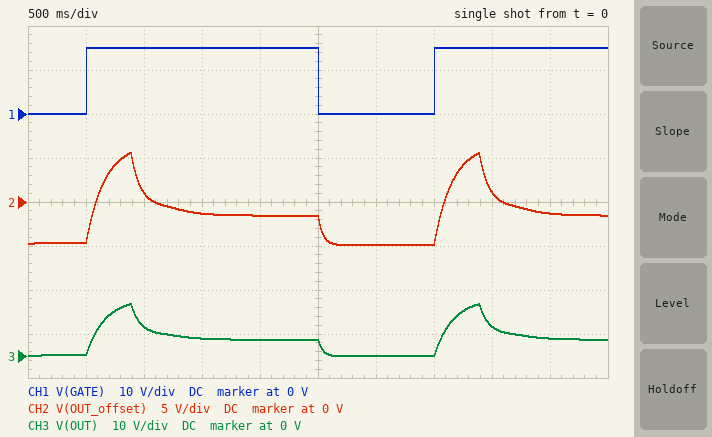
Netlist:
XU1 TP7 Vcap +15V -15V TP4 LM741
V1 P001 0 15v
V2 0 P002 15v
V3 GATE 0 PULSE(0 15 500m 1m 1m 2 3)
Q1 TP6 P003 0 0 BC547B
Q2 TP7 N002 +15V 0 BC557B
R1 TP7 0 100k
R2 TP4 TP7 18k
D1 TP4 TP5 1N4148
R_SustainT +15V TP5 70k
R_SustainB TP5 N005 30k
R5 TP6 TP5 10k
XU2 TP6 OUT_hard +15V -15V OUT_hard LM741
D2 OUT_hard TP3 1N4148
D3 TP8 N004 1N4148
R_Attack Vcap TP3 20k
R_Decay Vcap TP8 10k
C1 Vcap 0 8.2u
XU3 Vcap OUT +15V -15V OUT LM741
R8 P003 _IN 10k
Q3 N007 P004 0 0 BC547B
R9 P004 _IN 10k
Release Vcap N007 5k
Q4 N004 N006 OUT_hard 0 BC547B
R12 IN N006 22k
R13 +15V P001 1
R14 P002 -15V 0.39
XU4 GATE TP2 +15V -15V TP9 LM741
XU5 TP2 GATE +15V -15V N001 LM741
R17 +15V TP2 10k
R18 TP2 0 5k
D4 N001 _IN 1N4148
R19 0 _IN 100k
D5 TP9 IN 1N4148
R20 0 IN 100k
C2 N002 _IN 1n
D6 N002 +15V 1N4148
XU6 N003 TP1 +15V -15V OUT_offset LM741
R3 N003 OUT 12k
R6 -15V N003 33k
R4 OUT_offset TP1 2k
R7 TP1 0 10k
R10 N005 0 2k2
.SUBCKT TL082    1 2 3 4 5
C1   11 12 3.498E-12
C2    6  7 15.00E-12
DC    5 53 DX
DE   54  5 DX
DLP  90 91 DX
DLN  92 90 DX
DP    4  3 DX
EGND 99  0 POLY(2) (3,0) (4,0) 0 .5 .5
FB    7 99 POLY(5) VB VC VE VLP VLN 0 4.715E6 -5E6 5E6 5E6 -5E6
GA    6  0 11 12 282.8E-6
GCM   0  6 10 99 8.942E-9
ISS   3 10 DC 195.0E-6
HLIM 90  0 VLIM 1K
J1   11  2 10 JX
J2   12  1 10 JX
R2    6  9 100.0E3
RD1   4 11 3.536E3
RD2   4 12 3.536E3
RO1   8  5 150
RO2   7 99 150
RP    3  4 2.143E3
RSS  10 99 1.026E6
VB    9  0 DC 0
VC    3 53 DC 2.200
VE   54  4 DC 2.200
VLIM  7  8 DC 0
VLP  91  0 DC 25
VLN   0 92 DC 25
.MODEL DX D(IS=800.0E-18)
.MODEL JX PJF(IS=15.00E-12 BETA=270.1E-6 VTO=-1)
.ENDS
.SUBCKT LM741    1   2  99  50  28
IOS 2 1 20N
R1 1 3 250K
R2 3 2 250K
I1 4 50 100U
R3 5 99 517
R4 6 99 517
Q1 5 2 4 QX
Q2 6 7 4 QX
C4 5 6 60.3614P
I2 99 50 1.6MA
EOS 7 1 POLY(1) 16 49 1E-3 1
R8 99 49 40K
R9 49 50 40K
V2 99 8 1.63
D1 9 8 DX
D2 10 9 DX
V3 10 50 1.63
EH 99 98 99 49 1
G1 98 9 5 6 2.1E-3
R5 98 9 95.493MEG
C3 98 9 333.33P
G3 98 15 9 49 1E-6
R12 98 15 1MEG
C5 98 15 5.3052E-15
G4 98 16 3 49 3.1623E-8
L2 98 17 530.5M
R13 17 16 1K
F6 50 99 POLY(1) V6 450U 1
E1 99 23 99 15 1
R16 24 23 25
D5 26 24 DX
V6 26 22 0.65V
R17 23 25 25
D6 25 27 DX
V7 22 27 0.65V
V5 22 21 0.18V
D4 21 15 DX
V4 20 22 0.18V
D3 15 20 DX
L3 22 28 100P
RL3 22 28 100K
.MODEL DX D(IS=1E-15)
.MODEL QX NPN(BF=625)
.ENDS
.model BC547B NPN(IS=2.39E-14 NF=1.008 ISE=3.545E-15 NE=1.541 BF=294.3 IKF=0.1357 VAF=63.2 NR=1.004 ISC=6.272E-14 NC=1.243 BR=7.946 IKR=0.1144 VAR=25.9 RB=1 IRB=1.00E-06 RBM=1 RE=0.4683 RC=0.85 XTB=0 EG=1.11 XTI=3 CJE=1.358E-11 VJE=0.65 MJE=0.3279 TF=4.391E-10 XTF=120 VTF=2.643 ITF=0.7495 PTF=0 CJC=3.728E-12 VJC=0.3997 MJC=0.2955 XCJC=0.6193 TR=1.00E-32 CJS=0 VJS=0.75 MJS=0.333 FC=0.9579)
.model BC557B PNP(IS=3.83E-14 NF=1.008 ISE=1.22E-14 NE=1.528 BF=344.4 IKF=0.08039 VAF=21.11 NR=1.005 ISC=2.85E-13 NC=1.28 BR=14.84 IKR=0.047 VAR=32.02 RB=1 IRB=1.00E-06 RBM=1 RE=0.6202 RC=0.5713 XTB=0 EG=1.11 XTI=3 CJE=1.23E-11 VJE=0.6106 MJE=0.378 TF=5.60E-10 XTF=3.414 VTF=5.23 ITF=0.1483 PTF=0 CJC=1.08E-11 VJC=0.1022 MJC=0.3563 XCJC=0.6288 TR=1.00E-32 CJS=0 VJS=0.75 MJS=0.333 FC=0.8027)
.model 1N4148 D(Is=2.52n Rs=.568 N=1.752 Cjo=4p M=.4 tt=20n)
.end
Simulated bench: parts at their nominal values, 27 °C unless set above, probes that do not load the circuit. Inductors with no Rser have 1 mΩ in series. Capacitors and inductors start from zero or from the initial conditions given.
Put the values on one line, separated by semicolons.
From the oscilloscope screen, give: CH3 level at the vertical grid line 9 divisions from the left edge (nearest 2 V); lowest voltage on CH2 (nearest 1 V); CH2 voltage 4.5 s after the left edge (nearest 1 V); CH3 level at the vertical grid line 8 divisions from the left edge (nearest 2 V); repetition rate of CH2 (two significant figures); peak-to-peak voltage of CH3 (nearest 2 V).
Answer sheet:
4 V; -5 V; -1 V; 6 V; 330 mHz; 12 V
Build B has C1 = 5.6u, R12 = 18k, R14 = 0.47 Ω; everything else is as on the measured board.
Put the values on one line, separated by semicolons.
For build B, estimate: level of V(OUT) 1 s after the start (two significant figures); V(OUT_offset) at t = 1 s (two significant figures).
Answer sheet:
4.8 V; -610 mV
